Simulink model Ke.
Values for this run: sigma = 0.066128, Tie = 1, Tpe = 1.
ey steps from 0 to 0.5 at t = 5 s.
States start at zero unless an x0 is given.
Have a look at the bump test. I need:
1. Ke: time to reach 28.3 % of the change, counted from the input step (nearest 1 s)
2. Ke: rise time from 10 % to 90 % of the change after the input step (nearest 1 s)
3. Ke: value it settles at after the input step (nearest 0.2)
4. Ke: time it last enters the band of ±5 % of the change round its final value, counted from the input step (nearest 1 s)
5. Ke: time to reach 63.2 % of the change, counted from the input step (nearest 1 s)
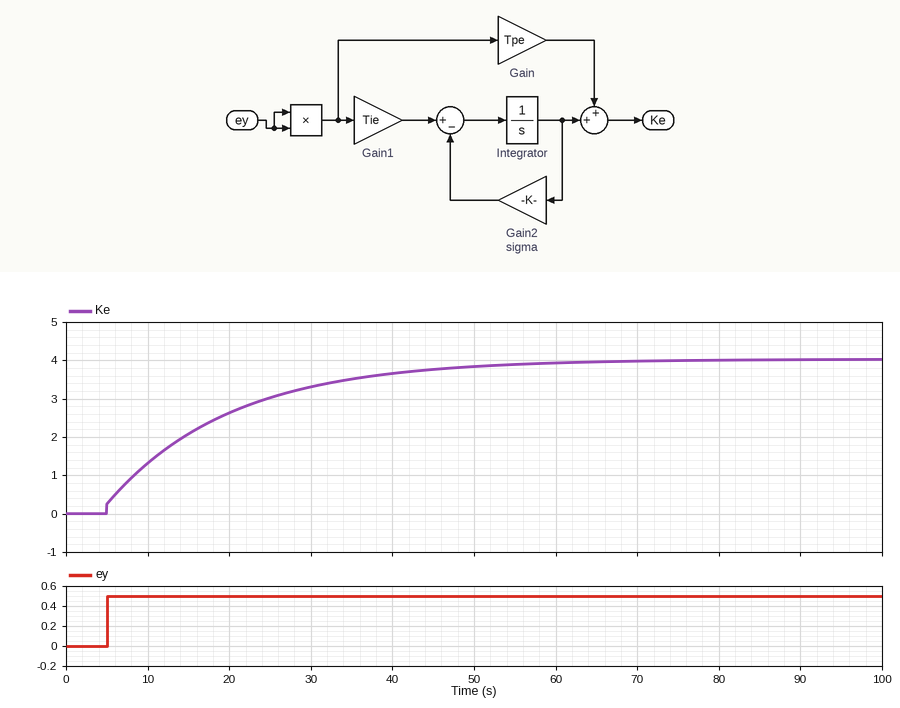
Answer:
4 s
33 s
4.0
44 s
14 s
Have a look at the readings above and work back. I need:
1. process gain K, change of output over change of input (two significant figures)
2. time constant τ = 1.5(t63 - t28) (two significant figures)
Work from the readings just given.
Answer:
8.0
15 s
